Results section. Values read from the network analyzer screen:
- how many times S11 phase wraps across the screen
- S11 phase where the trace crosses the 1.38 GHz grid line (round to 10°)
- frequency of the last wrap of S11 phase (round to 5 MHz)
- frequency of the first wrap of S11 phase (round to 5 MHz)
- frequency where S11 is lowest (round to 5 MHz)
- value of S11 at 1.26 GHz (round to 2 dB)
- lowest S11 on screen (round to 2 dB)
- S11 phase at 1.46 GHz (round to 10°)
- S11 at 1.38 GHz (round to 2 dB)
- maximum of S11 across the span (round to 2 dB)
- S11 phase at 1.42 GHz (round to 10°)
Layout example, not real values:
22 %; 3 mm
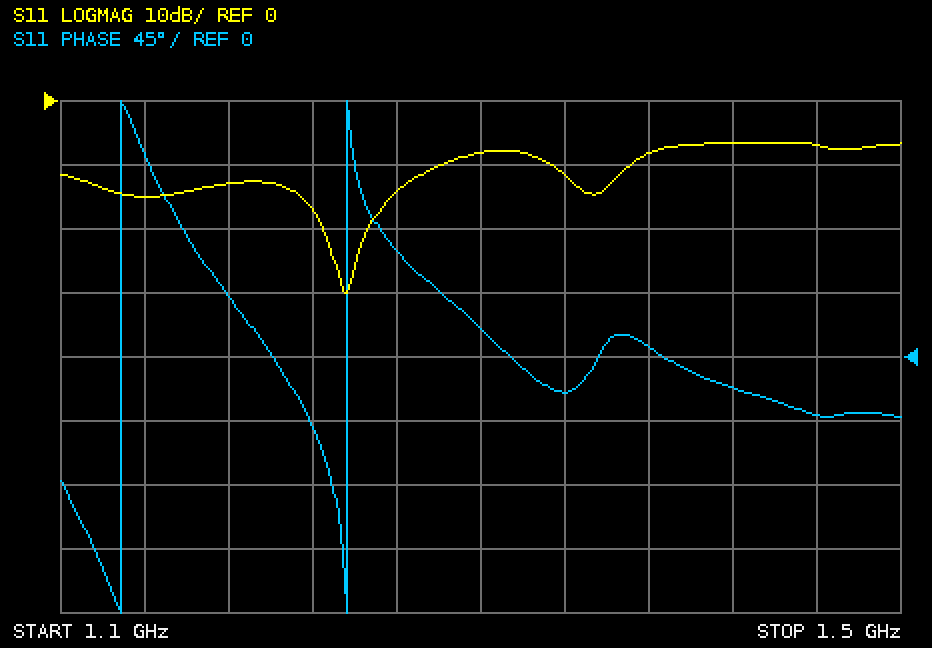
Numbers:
2; 10°; 1.235 GHz; 1.130 GHz; 1.235 GHz; -14 dB; -30 dB; -40°; -8 dB; -6 dB; -20°
